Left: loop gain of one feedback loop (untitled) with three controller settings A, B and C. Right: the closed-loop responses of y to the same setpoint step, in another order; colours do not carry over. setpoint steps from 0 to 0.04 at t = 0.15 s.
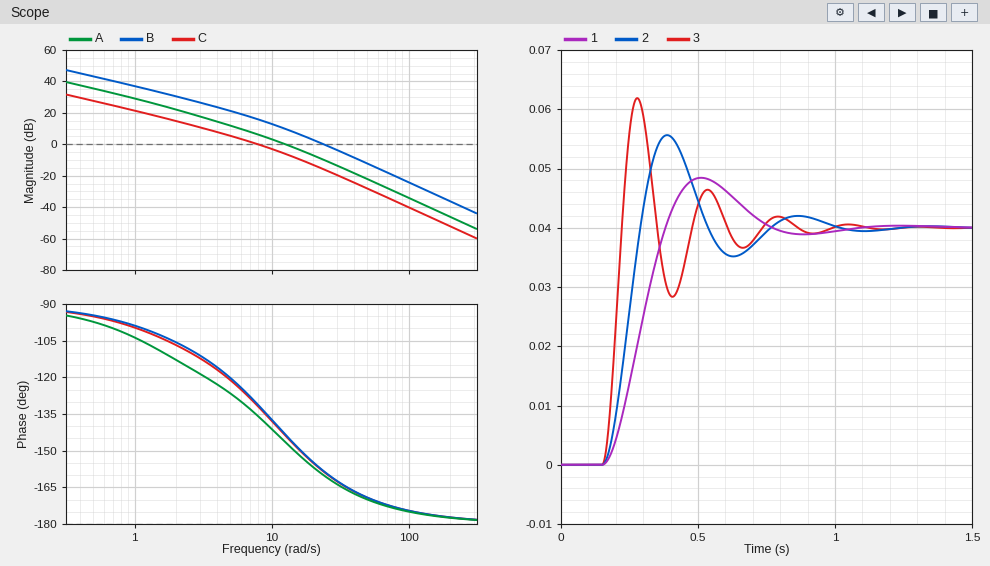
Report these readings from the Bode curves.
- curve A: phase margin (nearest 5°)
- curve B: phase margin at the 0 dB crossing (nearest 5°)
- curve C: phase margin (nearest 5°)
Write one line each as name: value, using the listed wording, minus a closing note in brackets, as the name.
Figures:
curve A: phase margin: 35°
curve B: phase margin at the 0 dB crossing: 20°
curve C: phase margin: 50°
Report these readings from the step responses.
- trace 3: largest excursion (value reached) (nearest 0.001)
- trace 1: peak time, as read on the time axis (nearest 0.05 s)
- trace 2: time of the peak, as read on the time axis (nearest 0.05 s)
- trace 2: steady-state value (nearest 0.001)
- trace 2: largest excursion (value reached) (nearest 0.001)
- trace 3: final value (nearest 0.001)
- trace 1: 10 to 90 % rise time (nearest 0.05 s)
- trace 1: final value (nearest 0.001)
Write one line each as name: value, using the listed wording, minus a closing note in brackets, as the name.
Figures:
trace 3: largest excursion (value reached): 0.062
trace 1: peak time, as read on the time axis: 0.50 s
trace 2: time of the peak, as read on the time axis: 0.40 s
trace 2: steady-state value: 0.040
trace 2: largest excursion (value reached): 0.056
trace 3: final value: 0.040
trace 1: 10 to 90 % rise time: 0.15 s
trace 1: final value: 0.040
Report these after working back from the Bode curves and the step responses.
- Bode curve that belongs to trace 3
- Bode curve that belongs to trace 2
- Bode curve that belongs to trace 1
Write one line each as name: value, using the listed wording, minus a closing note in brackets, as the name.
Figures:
Bode curve that belongs to trace 3: B
Bode curve that belongs to trace 2: A
Bode curve that belongs to trace 1: C
